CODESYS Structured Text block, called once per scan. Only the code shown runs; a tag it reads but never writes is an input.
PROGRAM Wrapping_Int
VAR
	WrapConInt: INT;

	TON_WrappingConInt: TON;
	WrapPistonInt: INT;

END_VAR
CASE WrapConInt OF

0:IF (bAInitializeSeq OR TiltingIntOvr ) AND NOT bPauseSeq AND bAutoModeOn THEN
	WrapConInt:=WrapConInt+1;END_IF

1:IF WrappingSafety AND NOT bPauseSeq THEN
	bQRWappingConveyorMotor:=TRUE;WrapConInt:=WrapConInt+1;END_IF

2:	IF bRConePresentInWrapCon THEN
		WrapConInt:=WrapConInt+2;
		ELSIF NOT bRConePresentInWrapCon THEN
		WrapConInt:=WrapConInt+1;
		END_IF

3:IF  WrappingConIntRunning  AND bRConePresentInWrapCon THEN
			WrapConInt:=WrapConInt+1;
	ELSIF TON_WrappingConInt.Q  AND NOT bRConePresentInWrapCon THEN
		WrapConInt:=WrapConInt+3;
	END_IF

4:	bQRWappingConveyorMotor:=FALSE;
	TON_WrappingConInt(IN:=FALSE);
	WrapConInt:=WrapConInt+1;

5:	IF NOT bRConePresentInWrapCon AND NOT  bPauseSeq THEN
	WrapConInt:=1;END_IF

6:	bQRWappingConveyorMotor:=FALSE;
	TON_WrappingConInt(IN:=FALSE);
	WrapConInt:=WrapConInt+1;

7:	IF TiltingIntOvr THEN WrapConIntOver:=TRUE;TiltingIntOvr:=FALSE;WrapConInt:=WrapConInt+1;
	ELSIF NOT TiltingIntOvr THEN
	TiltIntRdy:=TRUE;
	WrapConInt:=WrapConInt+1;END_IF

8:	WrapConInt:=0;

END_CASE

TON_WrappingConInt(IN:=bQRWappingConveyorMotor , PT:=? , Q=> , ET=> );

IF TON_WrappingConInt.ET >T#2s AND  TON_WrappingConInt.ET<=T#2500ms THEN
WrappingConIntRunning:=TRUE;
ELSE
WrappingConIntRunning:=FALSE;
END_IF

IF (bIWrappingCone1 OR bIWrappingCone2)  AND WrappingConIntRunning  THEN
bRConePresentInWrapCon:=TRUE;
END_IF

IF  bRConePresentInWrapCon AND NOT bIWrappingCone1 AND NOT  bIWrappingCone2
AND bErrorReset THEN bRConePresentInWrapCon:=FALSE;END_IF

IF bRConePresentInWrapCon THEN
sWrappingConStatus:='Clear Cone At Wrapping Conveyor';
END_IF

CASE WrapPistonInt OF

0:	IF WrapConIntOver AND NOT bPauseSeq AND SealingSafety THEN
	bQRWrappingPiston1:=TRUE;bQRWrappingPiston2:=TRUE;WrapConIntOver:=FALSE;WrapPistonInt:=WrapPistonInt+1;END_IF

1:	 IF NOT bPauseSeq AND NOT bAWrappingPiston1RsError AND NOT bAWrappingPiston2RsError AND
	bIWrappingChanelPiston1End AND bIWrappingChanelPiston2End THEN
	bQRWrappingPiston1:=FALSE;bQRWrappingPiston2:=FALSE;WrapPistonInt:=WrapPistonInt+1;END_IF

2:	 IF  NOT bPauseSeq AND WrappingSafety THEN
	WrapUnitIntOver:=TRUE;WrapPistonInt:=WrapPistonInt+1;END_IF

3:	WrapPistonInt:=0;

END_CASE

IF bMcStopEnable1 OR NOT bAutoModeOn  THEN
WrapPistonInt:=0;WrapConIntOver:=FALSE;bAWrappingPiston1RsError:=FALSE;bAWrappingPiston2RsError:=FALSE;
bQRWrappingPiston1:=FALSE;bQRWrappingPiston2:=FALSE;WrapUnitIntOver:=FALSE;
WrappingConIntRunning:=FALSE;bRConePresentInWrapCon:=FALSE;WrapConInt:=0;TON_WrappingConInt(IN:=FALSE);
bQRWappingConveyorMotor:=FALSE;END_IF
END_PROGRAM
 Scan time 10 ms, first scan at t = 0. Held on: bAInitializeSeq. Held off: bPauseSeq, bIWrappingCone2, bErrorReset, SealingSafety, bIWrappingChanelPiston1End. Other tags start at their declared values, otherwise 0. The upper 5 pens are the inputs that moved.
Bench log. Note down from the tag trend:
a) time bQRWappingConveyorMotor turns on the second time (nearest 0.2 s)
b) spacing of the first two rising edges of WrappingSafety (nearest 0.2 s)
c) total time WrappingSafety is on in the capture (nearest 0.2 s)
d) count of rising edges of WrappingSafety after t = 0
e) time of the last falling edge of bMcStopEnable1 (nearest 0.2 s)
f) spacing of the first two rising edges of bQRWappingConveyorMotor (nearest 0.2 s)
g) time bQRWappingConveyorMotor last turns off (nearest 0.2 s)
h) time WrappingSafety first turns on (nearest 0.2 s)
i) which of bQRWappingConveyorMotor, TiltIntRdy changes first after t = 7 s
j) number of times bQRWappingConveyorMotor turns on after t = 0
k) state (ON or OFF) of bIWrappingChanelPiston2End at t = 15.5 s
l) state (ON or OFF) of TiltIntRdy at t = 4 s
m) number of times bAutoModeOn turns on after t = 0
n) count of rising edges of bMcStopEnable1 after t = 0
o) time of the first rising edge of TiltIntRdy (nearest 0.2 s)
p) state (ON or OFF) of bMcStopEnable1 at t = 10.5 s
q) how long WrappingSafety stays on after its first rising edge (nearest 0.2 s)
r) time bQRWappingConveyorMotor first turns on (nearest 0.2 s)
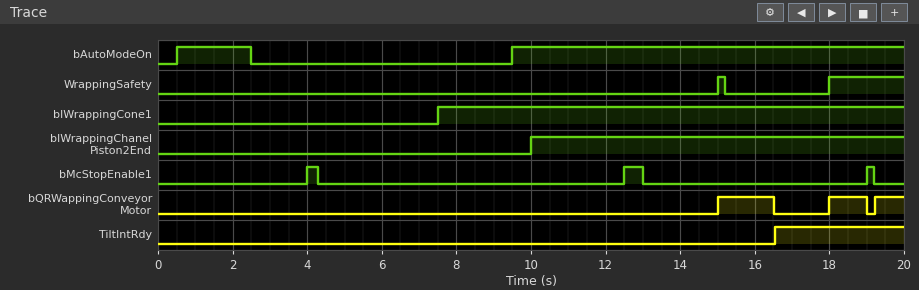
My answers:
18.0 s
3.0 s
2.2 s
2
19.2 s
3.0 s
19.0 s
15.0 s
bQRWappingConveyorMotor
3
ON
OFF
2
3
16.6 s
OFF
0.2 s
15.0 s
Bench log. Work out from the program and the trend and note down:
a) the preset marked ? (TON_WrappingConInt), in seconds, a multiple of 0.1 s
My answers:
1.5 s
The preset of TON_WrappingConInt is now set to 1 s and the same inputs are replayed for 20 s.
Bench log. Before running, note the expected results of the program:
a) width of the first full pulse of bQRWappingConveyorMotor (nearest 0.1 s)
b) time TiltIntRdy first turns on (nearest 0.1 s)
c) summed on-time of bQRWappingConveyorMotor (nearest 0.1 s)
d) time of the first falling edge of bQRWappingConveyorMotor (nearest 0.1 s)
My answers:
1.0 s
16.0 s
2.8 s
16.0 s
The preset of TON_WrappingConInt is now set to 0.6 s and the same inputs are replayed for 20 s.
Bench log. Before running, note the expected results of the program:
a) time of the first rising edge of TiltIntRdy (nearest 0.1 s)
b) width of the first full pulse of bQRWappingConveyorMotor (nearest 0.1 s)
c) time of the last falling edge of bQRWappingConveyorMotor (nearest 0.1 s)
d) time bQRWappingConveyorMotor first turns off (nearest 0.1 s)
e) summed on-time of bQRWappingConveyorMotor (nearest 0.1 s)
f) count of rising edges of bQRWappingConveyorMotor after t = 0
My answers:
15.6 s
0.6 s
19.8 s
15.6 s
2.3 s
5
